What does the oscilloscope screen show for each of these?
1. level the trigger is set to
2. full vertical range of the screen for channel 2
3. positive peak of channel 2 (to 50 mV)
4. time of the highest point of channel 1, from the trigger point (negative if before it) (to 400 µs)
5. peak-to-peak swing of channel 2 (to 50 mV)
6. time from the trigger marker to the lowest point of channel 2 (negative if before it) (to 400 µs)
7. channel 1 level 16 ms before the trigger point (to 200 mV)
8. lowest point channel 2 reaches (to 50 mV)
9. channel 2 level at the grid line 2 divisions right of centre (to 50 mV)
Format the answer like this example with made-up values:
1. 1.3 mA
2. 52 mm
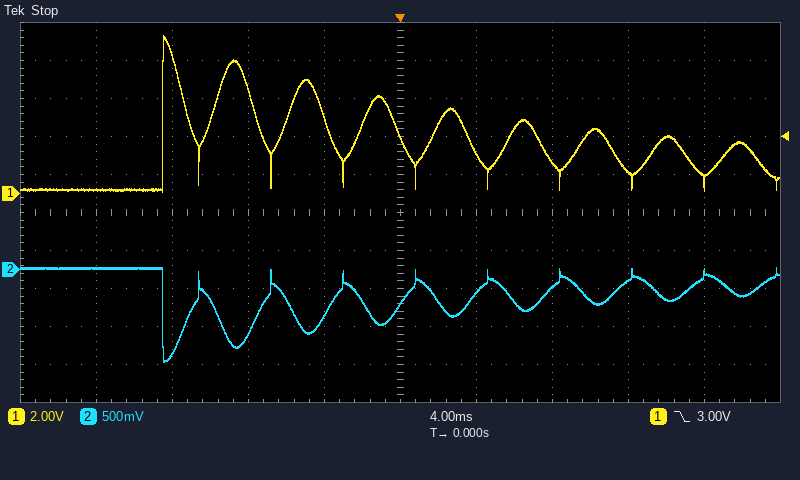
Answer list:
1. 3.00 V
2. 5 V
3. 50 mV
4. -12.4 ms
5. 1.25 V
6. -12.4 ms
7. 200 mV
8. -1.20 V
9. -250 mV
